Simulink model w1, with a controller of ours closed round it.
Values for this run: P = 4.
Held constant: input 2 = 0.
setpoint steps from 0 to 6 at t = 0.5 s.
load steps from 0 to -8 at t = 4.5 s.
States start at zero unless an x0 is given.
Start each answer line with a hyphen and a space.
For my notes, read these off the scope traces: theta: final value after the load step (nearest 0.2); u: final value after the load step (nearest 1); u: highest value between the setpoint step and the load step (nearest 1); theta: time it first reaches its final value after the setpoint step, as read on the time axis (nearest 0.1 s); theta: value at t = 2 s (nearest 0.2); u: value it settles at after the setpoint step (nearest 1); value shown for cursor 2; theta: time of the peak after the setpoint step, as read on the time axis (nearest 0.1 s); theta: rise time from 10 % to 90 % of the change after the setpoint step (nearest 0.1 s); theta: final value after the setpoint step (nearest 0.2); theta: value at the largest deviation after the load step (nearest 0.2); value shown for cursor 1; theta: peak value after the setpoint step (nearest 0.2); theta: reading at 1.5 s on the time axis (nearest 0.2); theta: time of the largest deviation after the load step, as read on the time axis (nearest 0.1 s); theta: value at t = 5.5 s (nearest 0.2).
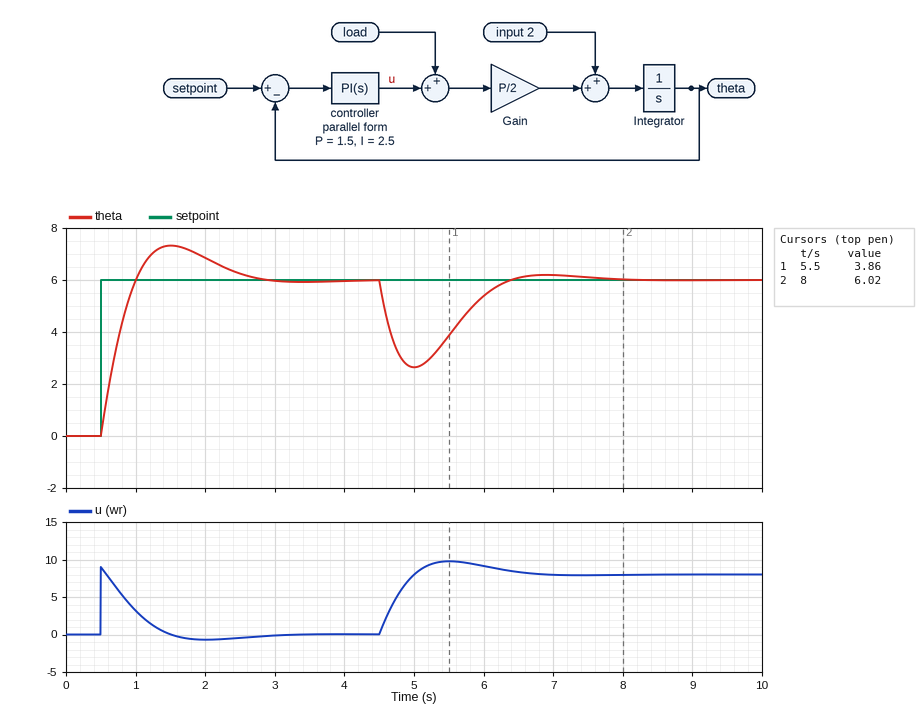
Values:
- 6.0
- 8
- 9
- 1.0 s
- 6.8
- 0
- 6.02
- 1.5 s
- 0.4 s
- 6.0
- 2.6
- 3.86
- 7.4
- 7.4
- 5.0 s
- 3.8
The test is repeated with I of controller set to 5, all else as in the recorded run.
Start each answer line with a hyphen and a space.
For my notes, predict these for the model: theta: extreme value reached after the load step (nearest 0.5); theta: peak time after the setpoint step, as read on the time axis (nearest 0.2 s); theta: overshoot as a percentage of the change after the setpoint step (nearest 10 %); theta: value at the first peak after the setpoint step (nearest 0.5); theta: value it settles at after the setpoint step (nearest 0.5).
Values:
- 3.0
- 1.2 s
- 30 %
- 8.0
- 6.0
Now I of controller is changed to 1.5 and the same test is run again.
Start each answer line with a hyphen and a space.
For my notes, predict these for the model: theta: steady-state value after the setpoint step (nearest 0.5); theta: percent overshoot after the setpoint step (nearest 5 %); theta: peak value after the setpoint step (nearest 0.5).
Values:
- 6.0
- 15 %
- 7.0
